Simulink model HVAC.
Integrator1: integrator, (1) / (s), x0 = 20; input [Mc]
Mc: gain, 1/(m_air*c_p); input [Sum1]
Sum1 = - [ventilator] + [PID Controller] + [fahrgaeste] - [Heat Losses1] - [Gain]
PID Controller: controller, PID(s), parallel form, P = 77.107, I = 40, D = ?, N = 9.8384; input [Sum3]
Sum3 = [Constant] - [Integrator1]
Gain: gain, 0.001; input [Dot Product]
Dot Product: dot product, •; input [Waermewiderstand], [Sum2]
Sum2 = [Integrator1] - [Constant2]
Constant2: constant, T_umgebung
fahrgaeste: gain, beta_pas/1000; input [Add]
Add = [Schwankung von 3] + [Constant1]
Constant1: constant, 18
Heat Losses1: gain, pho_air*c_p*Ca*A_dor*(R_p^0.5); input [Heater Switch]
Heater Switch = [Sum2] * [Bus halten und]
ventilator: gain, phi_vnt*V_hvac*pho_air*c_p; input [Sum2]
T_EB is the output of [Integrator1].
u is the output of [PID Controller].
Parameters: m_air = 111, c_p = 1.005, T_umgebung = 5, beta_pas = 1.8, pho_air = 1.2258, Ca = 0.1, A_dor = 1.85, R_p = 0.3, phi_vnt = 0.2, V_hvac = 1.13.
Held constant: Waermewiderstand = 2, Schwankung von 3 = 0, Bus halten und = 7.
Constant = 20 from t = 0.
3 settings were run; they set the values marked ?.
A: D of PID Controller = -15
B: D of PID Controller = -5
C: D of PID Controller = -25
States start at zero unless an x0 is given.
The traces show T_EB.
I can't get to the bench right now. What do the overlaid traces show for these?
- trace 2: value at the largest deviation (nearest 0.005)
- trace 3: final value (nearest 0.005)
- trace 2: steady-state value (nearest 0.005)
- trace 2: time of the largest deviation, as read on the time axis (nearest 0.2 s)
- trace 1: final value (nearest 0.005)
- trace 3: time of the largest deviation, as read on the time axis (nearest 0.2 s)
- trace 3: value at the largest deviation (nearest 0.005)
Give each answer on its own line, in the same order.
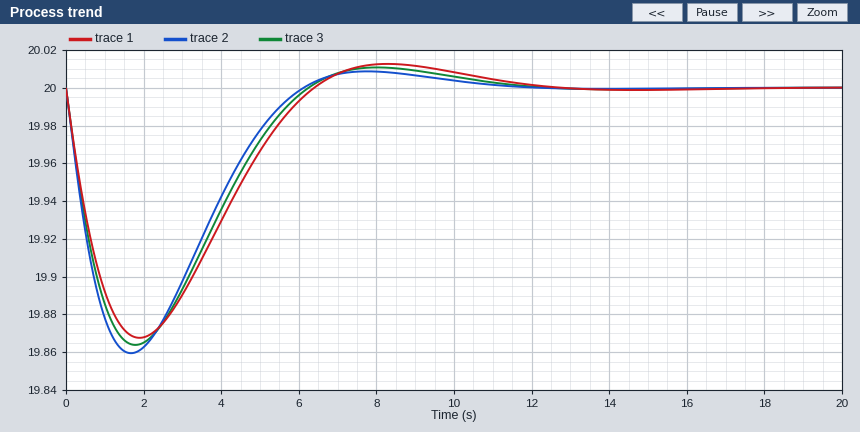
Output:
19.860
20.000
20.000
1.6 s
20.000
1.8 s
19.865
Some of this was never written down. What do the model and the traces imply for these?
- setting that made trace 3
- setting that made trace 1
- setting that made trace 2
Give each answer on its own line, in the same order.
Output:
A
B
C
